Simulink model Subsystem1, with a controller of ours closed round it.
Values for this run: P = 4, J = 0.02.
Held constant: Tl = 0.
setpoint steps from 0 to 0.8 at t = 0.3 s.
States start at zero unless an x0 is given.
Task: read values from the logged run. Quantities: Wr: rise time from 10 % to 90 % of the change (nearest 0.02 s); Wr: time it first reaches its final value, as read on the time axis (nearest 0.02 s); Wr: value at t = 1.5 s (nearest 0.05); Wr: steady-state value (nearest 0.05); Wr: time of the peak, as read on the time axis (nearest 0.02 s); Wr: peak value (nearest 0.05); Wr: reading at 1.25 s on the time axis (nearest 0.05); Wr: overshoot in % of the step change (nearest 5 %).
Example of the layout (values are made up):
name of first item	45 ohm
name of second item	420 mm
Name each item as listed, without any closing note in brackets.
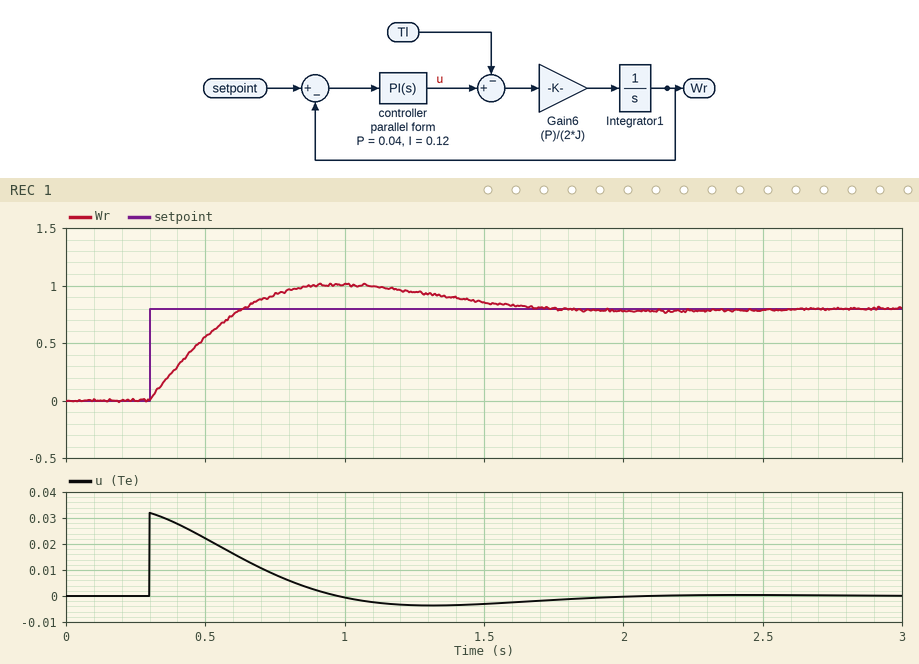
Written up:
Wr: rise time from 10 % to 90 % of the change	0.26 s
Wr: time it first reaches its final value, as read on the time axis	0.64 s
Wr: value at t = 1.5 s	0.85
Wr: steady-state value	0.80
Wr: time of the peak, as read on the time axis	0.98 s
Wr: peak value	1.00
Wr: reading at 1.25 s on the time axis	0.95
Wr: overshoot in % of the step change	25 %
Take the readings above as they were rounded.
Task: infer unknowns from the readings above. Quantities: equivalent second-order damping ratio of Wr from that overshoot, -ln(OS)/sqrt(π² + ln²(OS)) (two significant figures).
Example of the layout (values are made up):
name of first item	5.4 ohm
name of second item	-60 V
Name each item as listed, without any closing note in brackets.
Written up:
equivalent second-order damping ratio of Wr from that overshoot, -ln(OS)/sqrt(π² + ln²(OS))	0.40
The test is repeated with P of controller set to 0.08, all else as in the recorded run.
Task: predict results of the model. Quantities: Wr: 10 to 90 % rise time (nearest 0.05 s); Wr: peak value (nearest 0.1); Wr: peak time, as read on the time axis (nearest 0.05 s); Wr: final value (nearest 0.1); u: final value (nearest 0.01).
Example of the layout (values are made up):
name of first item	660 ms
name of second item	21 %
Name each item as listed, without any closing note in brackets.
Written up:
Wr: 10 to 90 % rise time	0.20 s
Wr: peak value	0.9
Wr: peak time, as read on the time axis	0.85 s
Wr: final value	0.8
u: final value	0.00
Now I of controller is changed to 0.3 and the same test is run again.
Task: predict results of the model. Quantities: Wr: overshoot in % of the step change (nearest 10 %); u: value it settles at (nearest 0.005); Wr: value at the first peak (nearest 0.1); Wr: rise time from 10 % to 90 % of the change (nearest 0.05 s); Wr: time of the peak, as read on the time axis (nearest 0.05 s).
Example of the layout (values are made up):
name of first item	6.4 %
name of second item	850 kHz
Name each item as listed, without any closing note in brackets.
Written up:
Wr: overshoot in % of the step change	40 %
u: value it settles at	0.000
Wr: value at the first peak	1.1
Wr: rise time from 10 % to 90 % of the change	0.20 s
Wr: time of the peak, as read on the time axis	0.75 s
